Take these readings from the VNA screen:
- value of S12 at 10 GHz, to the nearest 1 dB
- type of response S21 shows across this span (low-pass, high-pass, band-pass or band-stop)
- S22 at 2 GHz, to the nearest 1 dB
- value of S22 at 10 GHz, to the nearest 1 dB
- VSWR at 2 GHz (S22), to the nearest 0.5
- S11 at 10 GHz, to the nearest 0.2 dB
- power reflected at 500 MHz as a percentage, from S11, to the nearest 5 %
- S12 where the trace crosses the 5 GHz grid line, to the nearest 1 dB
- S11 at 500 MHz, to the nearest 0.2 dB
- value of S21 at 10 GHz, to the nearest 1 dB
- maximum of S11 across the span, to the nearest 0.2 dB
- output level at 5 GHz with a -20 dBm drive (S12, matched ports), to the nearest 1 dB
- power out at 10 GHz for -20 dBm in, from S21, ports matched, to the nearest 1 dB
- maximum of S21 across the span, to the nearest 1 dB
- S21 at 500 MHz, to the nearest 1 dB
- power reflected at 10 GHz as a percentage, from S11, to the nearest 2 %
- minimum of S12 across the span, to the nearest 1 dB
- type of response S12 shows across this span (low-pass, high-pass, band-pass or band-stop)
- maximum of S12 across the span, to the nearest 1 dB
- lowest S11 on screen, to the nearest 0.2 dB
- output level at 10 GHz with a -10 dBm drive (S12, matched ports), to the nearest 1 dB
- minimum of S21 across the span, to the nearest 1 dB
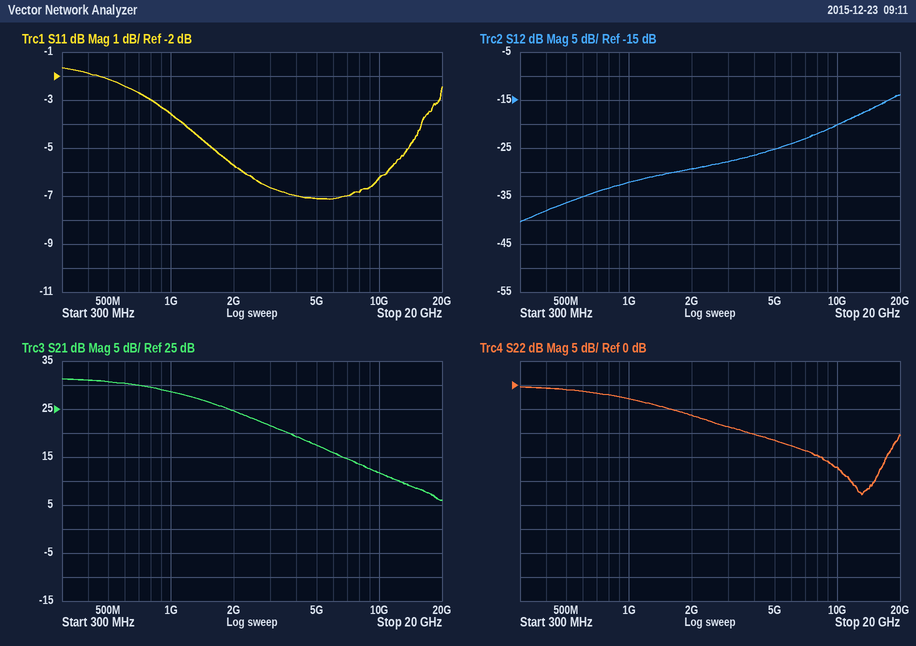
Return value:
-20 dB
low-pass
-6 dB
-17 dB
3.0
-6.2 dB
60 %
-25 dB
-2.2 dB
12 dB
-1.6 dB
-45 dBm
-8 dBm
31 dB
31 dB
24 %
-40 dB
high-pass
-14 dB
-7.2 dB
-30 dBm
6 dB
